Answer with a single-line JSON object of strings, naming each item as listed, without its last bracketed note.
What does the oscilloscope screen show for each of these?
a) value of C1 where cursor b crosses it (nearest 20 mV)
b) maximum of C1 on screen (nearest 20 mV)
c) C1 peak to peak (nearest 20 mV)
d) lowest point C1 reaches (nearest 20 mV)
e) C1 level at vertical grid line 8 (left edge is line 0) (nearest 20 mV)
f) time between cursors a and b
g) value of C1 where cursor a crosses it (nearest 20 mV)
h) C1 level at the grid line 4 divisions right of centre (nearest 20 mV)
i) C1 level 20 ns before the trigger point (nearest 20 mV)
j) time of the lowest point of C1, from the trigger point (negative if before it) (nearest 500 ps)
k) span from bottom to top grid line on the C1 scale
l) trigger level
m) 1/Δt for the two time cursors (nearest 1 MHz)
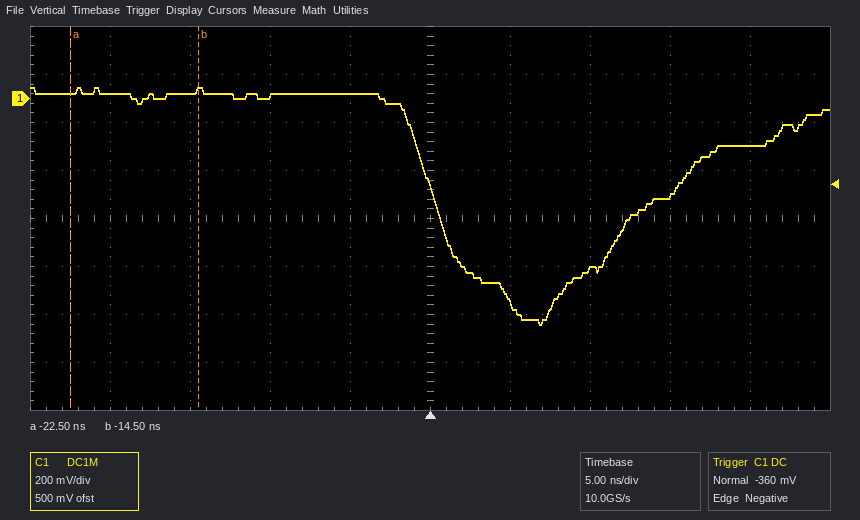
{"value of C1 where cursor b crosses it": "40 mV", "maximum of C1 on screen": "40 mV", "C1 peak to peak": "980 mV", "lowest point C1 reaches": "-940 mV", "C1 level at vertical grid line 8 (left edge is line 0)": "-400 mV", "time between cursors a and b": "8.0 ns", "value of C1 where cursor a crosses it": "20 mV", "C1 level at the grid line 4 divisions right of centre": "-200 mV", "C1 level 20 ns before the trigger point": "20 mV", "time of the lowest point of C1, from the trigger point (negative if before it)": "+7.0 ns", "span from bottom to top grid line on the C1 scale": "1.6 V", "trigger level": "-360 mV", "1/Δt for the two time cursors": "125 MHz"}
